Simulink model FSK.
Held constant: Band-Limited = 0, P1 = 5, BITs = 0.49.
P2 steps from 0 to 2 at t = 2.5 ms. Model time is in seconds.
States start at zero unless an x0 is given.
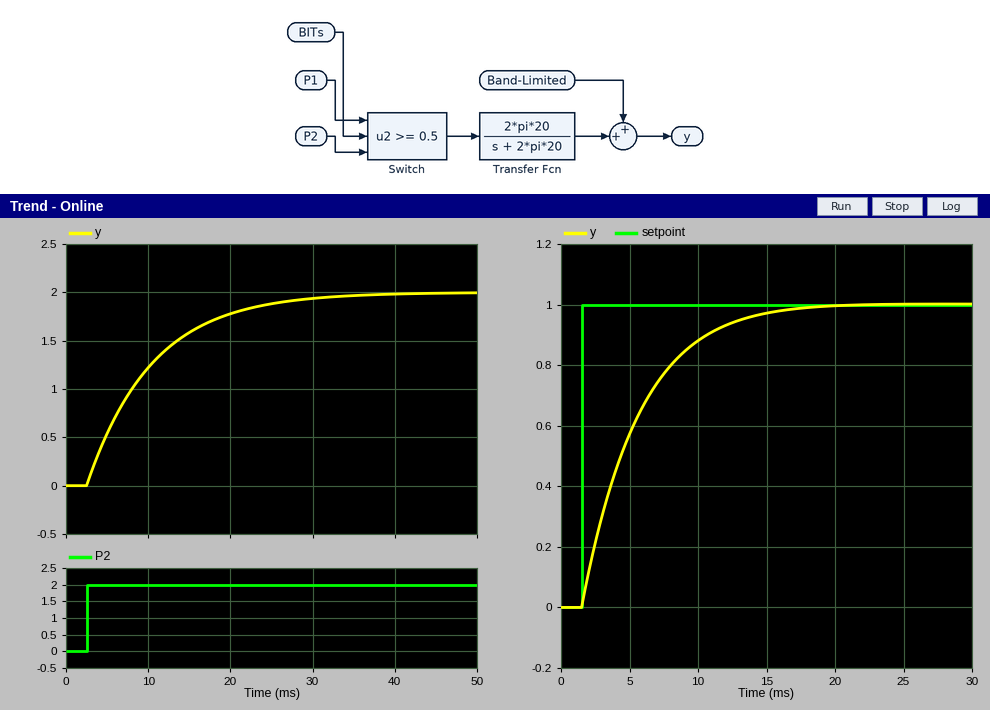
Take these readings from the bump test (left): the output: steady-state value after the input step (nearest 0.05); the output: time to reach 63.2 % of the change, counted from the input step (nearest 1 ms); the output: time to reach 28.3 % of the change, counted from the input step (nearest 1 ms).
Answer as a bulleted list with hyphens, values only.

- 2.00
- 8 ms
- 3 ms
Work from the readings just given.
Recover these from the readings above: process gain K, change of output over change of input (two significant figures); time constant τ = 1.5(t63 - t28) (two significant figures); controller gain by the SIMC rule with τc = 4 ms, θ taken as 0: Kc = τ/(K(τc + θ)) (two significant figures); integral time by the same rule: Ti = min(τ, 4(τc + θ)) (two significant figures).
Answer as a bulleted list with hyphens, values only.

- 1.0
- 7.5 ms
- 1.9
- 7.5 ms
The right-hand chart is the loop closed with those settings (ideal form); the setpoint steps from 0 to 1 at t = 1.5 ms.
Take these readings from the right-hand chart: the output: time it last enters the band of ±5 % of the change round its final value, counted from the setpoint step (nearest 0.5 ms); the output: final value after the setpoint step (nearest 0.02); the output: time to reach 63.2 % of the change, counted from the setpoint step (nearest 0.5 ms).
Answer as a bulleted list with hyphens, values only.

- 11.5 ms
- 1.00
- 4.0 ms
